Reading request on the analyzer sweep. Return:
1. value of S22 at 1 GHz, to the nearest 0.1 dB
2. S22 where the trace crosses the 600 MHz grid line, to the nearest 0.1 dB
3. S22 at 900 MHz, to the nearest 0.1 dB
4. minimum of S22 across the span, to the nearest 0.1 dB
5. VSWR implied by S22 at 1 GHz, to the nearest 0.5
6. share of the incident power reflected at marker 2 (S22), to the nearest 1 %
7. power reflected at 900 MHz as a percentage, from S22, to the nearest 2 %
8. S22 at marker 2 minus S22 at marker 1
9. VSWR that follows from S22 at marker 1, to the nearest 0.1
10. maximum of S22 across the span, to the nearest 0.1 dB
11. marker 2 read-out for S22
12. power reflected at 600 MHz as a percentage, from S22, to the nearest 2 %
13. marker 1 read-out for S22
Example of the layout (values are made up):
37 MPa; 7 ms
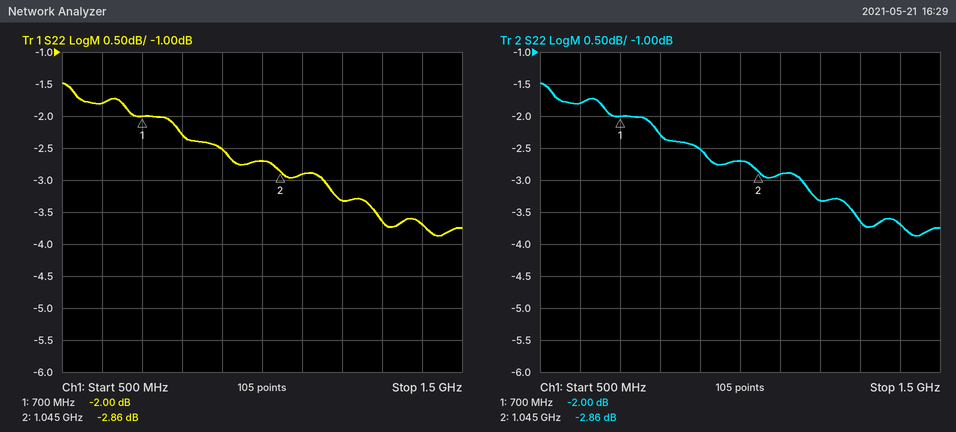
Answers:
-2.7 dB; -1.8 dB; -2.5 dB; -3.9 dB; 6.5; 52 %; 56 %; -0.86 dB; 8.7; -1.5 dB; -2.86 dB; 66 %; -2.00 dB
